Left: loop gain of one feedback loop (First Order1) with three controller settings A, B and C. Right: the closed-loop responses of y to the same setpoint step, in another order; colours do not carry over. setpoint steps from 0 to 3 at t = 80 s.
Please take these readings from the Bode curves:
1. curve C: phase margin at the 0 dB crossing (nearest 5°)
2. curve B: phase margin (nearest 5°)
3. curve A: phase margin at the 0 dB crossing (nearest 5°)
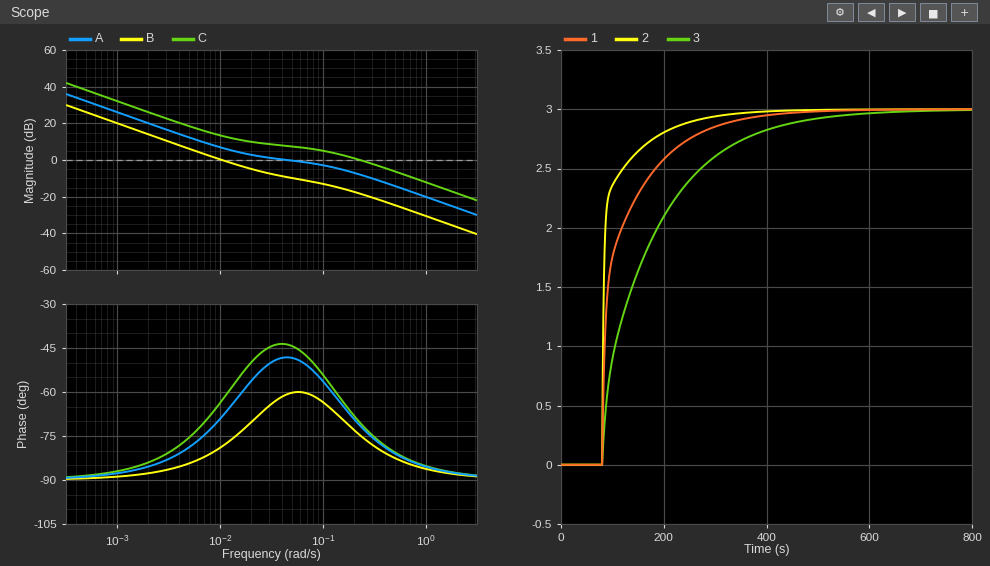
110°
100°
130°
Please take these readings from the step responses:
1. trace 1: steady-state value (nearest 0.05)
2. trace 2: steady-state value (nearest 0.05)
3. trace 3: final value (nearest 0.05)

3.00
3.00
3.00
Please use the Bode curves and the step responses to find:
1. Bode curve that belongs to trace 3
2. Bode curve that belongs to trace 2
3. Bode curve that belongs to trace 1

B
C
A
